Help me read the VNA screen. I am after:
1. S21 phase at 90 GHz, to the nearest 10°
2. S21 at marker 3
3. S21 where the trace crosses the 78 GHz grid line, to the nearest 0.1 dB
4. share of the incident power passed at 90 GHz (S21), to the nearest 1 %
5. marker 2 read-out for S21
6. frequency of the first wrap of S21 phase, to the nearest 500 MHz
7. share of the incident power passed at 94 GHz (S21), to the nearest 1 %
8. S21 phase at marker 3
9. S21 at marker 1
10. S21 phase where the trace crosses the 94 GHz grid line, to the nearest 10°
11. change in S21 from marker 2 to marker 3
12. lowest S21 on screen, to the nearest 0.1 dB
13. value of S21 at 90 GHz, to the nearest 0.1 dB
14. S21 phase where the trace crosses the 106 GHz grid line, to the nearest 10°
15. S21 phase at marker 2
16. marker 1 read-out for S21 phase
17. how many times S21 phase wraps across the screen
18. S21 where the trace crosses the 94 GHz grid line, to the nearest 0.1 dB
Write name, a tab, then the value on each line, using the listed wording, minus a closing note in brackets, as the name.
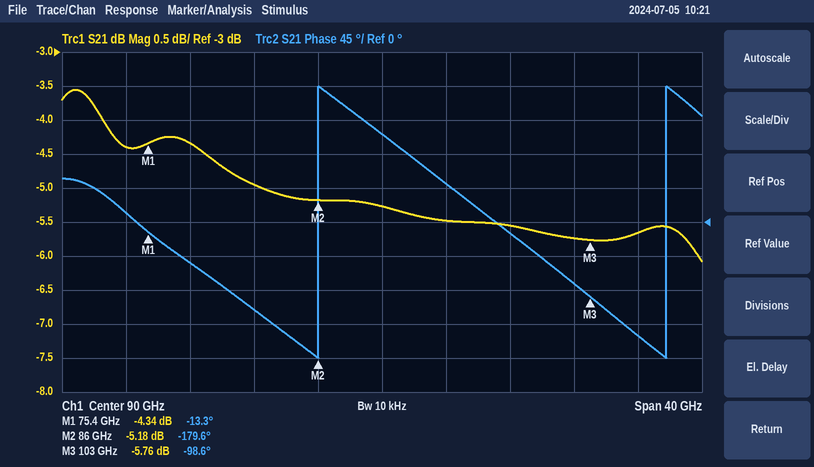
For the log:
S21 phase at 90 GHz, to the nearest 10°	120°
S21 at marker 3	-5.76 dB
S21 where the trace crosses the 78 GHz grid line, to the nearest 0.1 dB	-4.3 dB
share of the incident power passed at 90 GHz (S21), to the nearest 1 %	30 %
marker 2 read-out for S21	-5.18 dB
frequency of the first wrap of S21 phase, to the nearest 500 MHz	86.0 GHz
share of the incident power passed at 94 GHz (S21), to the nearest 1 %	28 %
S21 phase at marker 3	-98.6°
S21 at marker 1	-4.34 dB
S21 phase where the trace crosses the 94 GHz grid line, to the nearest 10°	50°
change in S21 from marker 2 to marker 3	-0.58 dB
lowest S21 on screen, to the nearest 0.1 dB	-6.1 dB
value of S21 at 90 GHz, to the nearest 0.1 dB	-5.3 dB
S21 phase where the trace crosses the 106 GHz grid line, to the nearest 10°	-150°
S21 phase at marker 2	-179.6°
marker 1 read-out for S21 phase	-13.3°
how many times S21 phase wraps across the screen	2
S21 where the trace crosses the 94 GHz grid line, to the nearest 0.1 dB	-5.5 dB
